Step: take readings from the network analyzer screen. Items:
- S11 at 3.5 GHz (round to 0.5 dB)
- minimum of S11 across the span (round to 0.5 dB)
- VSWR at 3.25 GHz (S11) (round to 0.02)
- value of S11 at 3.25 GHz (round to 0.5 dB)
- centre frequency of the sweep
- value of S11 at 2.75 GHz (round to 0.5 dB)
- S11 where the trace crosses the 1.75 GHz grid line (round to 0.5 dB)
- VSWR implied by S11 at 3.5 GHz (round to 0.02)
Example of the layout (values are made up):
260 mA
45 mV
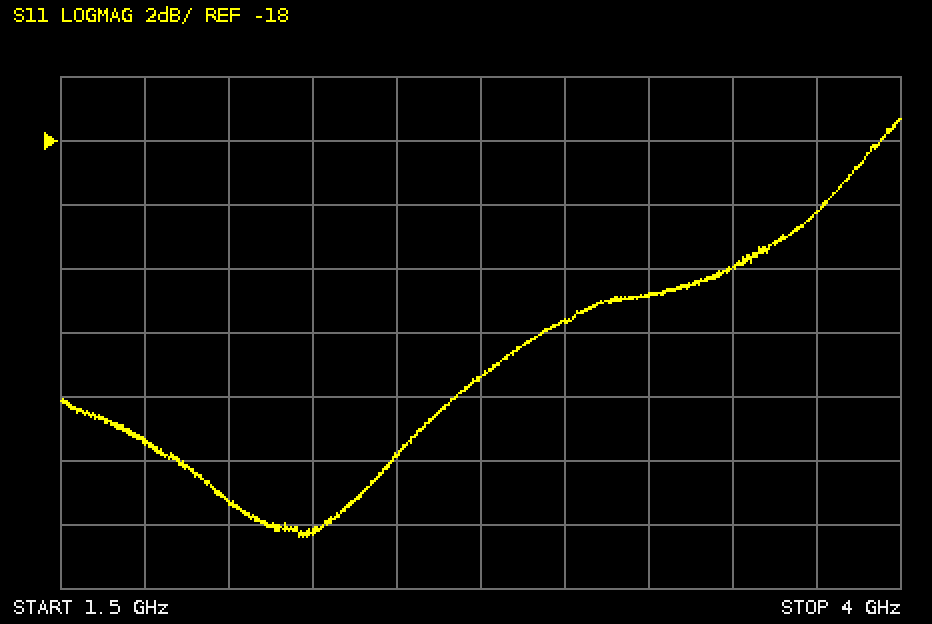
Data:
-22.0 dB
-30.5 dB
1.16
-23.0 dB
2.75 GHz
-25.5 dB
-27.5 dB
1.18
